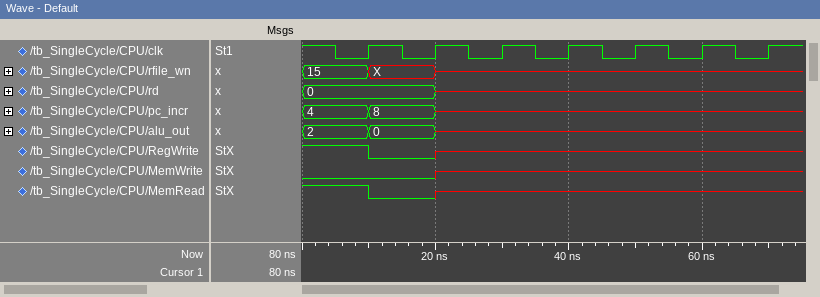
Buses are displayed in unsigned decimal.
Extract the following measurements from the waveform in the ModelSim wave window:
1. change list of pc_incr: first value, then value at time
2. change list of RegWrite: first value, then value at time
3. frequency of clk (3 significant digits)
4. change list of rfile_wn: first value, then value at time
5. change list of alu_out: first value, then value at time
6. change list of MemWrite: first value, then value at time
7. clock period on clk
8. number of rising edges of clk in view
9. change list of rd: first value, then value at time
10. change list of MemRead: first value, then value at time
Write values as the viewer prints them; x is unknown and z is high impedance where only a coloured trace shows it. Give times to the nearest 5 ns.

4, 8 at 10 ns, x at 20 ns
1, 0 at 10 ns, x at 20 ns
100 MHz
15, X at 10 ns, x at 20 ns
2, 0 at 10 ns, x at 20 ns
0, x at 20 ns
10 ns
7
0, x at 20 ns
1, 0 at 10 ns, x at 20 ns
